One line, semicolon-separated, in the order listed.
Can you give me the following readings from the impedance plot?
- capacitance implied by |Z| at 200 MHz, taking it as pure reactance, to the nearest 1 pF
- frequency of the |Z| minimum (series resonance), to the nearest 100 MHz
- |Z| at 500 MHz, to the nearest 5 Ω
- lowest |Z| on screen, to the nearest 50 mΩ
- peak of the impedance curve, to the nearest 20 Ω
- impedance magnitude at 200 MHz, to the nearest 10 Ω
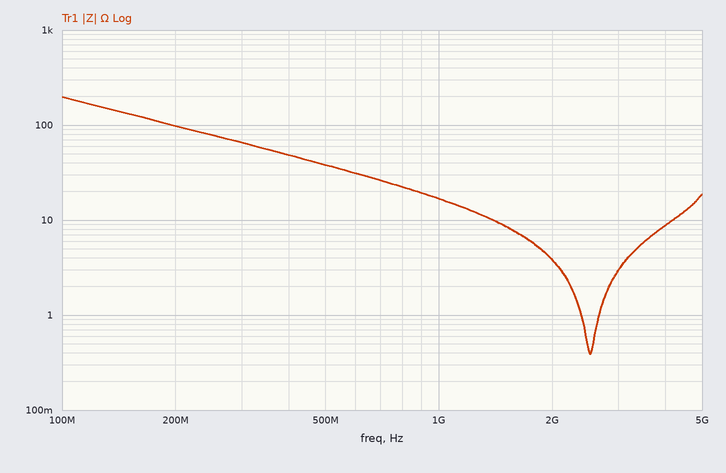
8 pF; 2.5 GHz; 40 Ω; 400 mΩ; 200 Ω; 100 Ω
